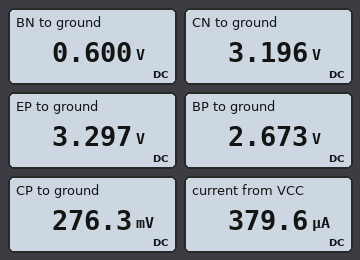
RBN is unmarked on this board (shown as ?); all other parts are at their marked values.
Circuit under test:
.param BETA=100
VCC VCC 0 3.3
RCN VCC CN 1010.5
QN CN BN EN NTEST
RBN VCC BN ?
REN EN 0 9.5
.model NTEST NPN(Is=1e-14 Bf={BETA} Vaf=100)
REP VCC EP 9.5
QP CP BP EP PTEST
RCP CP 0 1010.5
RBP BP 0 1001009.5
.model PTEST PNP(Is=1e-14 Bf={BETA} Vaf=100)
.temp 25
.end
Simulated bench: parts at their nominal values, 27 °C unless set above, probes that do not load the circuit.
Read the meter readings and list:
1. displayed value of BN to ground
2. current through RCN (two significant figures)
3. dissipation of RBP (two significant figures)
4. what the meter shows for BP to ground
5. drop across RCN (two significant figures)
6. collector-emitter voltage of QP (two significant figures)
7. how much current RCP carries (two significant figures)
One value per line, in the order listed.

0.600 V
100 µA
7.1 µW
2.673 V
100 mV
-3.0 V
270 µA
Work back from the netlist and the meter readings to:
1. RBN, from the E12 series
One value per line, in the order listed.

2.7 MΩ
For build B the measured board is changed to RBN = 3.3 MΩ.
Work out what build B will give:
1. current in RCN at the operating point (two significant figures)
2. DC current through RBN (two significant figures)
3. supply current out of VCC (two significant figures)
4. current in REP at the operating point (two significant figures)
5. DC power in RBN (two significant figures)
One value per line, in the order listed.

84 µA
820 nA
360 µA
280 µA
2.2 µW
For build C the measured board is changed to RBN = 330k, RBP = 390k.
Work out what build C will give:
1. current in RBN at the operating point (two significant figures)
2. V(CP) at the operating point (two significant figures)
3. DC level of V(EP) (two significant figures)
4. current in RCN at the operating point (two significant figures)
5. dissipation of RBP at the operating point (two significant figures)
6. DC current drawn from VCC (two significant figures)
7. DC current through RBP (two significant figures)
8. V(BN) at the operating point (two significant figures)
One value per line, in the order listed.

8.0 µA
700 mV
3.3 V
810 µA
18 µW
1.5 mA
6.8 µA
660 mV
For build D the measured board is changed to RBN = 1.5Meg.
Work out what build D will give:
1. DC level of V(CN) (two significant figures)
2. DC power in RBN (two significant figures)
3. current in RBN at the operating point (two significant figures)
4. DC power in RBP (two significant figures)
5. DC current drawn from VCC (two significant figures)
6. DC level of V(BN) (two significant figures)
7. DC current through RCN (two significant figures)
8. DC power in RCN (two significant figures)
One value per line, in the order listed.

3.1 V
4.8 µW
1.8 µA
7.1 µW
460 µA
620 mV
180 µA
34 µW
